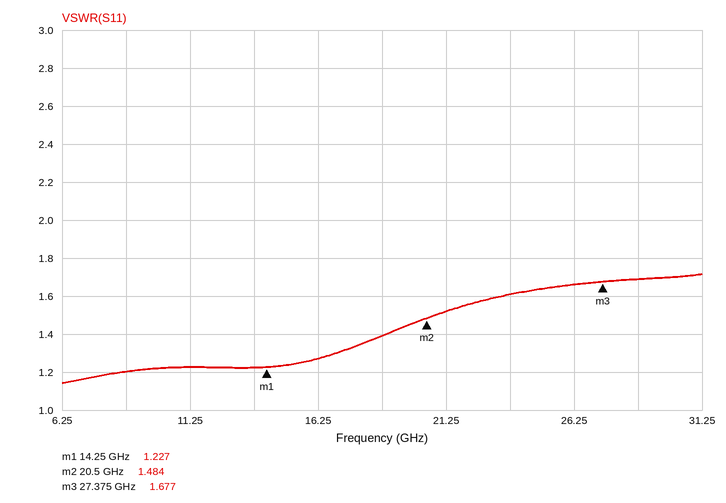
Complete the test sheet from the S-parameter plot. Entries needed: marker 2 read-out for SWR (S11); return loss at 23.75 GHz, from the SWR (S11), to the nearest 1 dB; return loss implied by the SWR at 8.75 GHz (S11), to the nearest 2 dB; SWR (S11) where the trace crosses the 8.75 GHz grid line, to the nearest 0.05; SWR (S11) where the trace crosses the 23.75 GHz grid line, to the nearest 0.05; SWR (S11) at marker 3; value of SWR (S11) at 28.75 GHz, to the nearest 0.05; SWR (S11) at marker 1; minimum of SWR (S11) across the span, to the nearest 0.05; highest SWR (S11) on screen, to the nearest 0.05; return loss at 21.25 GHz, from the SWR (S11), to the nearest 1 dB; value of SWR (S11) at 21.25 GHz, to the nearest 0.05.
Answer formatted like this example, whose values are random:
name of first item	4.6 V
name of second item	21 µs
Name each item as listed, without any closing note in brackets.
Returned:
marker 2 read-out for SWR	1.484
return loss at 23.75 GHz, from the SWR (S11), to the nearest 1 dB	13 dB
return loss implied by the SWR at 8.75 GHz (S11), to the nearest 2 dB	20 dB
SWR (S11) where the trace crosses the 8.75 GHz grid line, to the nearest 0.05	1.20
SWR (S11) where the trace crosses the 23.75 GHz grid line, to the nearest 0.05	1.60
SWR (S11) at marker 3	1.677
value of SWR (S11) at 28.75 GHz, to the nearest 0.05	1.70
SWR (S11) at marker 1	1.227
minimum of SWR (S11) across the span, to the nearest 0.05	1.15
highest SWR (S11) on screen, to the nearest 0.05	1.70
return loss at 21.25 GHz, from the SWR (S11), to the nearest 1 dB	14 dB
value of SWR (S11) at 21.25 GHz, to the nearest 0.05	1.50
